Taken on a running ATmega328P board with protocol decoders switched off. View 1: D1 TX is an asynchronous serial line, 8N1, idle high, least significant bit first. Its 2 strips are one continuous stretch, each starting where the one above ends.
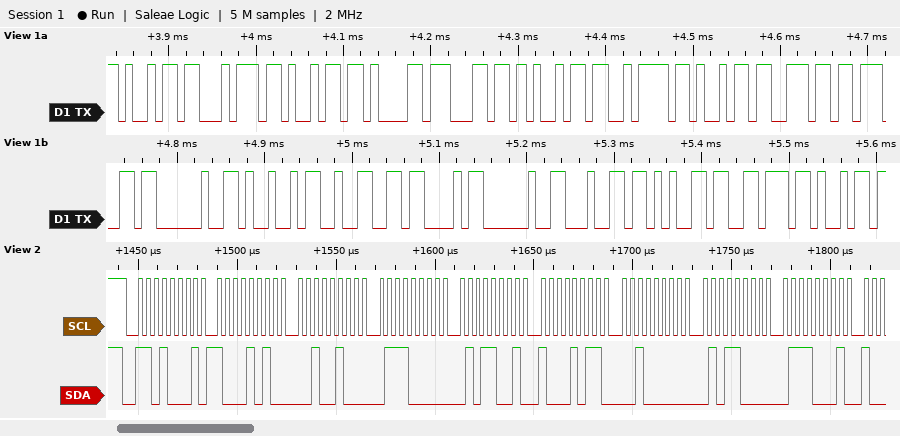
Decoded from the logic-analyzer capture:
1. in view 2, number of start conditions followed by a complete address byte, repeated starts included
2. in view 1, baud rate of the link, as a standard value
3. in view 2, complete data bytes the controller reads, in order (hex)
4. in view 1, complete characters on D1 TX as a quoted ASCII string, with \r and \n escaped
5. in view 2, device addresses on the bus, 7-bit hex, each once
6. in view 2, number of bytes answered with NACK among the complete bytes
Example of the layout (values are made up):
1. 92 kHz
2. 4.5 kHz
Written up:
1. 1
2. 115200 baud
3. 8A 24 70 59 8B 20 58 71
4. "itializing I2C devi"
5. 0x68
6. 0
